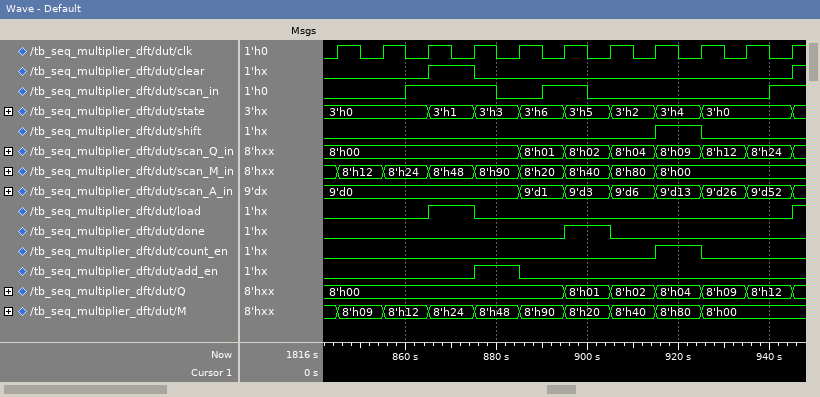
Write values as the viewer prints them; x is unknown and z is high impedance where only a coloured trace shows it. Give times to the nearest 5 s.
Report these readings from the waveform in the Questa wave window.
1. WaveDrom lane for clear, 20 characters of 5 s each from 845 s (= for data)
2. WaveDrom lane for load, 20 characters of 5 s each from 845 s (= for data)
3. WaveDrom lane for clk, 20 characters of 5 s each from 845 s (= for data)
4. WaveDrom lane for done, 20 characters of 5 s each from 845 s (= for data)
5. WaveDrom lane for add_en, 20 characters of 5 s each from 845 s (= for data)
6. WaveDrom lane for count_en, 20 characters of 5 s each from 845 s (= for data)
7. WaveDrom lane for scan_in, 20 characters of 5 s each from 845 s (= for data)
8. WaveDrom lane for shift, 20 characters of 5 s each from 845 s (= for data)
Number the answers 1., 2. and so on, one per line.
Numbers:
1. {name: 'clear', wave: '0...1.0.............'}
2. {name: 'load', wave: '0...1.0.............'}
3. {name: 'clk', wave: '10101010101010101010'}
4. {name: 'done', wave: '0.........1.0.......'}
5. {name: 'add_en', wave: '0.....1.0...........'}
6. {name: 'count_en', wave: '0.............1.0...'}
7. {name: 'scan_in', wave: '0..1...0.1.0.......1'}
8. {name: 'shift', wave: '0.............1.0...'}
